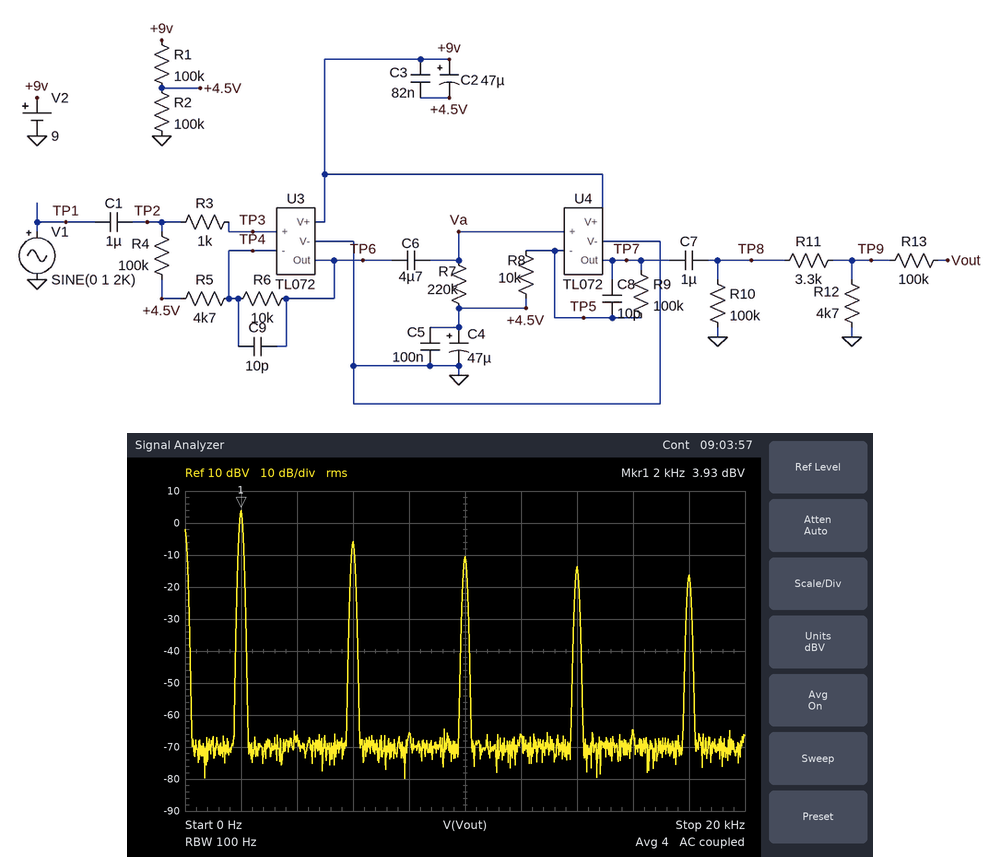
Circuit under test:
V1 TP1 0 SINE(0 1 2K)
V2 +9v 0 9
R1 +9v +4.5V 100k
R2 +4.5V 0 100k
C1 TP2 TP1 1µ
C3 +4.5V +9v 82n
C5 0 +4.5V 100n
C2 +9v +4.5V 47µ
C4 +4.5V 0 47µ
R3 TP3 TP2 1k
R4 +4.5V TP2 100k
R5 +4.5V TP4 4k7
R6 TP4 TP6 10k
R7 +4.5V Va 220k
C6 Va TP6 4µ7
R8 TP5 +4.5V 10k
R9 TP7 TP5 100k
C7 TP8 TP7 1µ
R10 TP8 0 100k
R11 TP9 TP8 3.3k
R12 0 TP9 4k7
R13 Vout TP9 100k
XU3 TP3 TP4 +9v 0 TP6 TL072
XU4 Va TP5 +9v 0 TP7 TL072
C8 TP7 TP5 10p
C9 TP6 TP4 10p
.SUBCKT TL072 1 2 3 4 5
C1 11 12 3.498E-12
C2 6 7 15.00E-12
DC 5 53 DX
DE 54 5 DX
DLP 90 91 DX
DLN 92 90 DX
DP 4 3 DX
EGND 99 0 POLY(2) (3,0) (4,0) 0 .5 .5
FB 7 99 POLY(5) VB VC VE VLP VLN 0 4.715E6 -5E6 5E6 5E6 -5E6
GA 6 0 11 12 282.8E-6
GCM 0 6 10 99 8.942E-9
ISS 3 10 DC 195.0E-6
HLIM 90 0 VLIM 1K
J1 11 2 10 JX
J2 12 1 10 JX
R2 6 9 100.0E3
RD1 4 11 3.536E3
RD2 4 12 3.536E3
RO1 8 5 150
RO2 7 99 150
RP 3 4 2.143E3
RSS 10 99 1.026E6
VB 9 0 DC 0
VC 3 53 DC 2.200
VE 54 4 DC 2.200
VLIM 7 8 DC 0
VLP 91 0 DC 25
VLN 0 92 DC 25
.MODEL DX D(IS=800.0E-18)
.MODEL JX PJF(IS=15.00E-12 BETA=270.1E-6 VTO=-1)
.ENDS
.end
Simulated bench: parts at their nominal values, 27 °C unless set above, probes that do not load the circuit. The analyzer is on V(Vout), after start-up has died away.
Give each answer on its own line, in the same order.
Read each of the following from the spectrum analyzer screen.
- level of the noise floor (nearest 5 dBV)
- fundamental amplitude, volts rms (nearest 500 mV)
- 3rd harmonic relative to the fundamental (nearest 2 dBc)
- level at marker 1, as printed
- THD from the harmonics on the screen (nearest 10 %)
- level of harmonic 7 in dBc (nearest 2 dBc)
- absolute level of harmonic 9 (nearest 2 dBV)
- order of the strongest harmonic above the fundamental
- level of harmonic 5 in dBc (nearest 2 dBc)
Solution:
-70 dBV
1.5 V
-10 dBc
3.93 dBV
40 %
-18 dBc
-16 dBV
3
-14 dBc
